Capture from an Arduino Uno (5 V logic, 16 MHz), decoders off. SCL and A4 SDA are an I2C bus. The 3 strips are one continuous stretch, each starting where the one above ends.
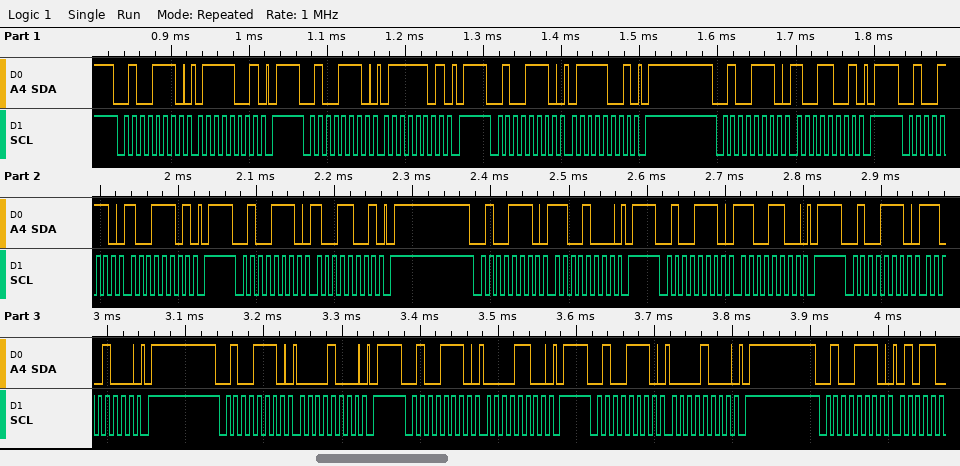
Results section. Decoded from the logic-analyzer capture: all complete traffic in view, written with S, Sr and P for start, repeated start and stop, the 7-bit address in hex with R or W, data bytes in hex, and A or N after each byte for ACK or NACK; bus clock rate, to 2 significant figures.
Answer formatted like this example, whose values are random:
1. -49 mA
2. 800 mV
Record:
1. S 27W A 79 A P S 27W A 7D A P S 27W A 79 A P S 27W A 99 A P S 27W A 9D A P S 27W A 99 A P S 27W A C8 A P S 27W A CC A P S 27W A C8 A P S 27W A 08 A P S 27W A 0C A P S 27W A 08 A P S 27W A
2. 100 kHz
